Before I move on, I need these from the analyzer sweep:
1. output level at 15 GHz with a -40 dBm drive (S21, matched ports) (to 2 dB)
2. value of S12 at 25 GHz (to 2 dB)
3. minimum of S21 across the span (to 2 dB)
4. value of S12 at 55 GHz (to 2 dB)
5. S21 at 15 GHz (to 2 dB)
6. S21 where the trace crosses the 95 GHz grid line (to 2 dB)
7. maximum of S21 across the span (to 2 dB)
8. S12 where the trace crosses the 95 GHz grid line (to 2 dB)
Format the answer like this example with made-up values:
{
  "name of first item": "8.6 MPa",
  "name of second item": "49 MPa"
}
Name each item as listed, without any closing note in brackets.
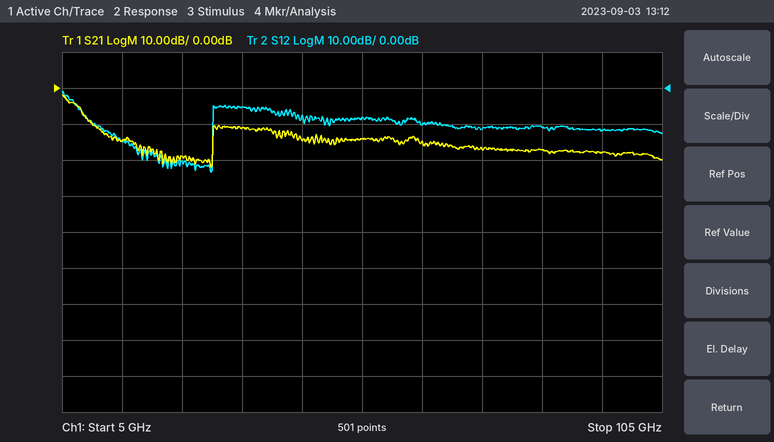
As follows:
{
  "output level at 15 GHz with a -40 dBm drive (S21, matched ports)": "-54 dBm",
  "value of S12 at 25 GHz": "-20 dB",
  "minimum of S21 across the span": "-22 dB",
  "value of S12 at 55 GHz": "-8 dB",
  "S21 at 15 GHz": "-14 dB",
  "S21 where the trace crosses the 95 GHz grid line": "-18 dB",
  "maximum of S21 across the span": "-2 dB",
  "S12 where the trace crosses the 95 GHz grid line": "-12 dB"
}
